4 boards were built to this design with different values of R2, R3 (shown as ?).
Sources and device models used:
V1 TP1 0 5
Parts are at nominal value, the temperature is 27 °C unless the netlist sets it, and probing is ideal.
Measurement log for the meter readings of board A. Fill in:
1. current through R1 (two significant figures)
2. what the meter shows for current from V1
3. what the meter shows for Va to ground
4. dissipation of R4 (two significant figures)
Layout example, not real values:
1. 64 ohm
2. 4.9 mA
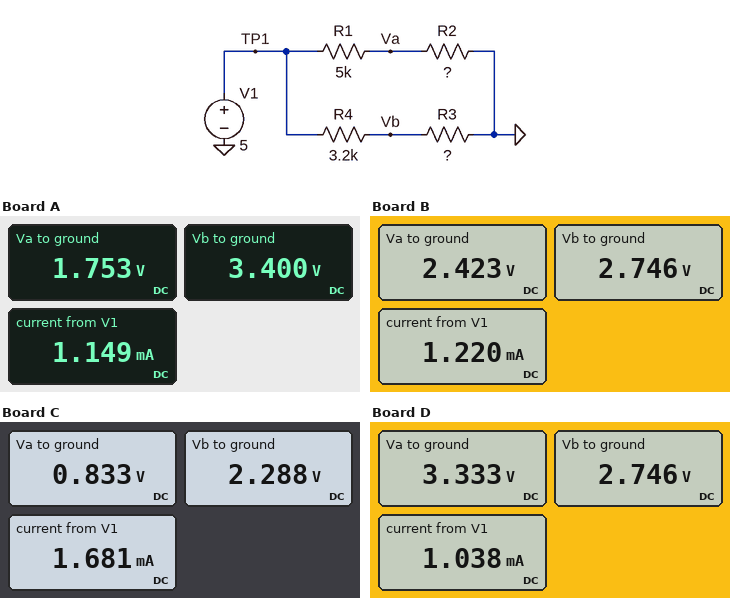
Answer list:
1. 650 µA
2. 1.149 mA
3. 1.753 V
4. 800 µW
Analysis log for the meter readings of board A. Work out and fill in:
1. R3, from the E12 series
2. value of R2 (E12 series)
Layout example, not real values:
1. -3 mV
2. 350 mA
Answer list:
1. 6.8 kΩ
2. 2.7 kΩ
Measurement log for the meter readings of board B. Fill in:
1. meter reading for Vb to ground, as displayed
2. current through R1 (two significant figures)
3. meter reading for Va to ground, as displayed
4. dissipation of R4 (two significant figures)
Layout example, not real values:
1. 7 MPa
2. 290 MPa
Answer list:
1. 2.746 V
2. 520 µA
3. 2.423 V
4. 1.6 mW
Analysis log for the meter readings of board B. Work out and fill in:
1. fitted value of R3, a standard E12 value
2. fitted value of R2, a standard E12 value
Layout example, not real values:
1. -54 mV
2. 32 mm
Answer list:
1. 3.9 kΩ
2. 4.7 kΩ
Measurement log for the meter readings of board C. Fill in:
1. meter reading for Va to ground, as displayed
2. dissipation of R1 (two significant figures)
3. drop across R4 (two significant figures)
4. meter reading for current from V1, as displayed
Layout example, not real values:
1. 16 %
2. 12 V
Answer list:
1. 0.833 V
2. 3.5 mW
3. 2.7 V
4. 1.681 mA
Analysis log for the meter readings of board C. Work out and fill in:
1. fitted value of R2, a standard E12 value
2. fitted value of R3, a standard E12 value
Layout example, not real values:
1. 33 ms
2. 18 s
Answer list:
1. 1 kΩ
2. 2.7 kΩ
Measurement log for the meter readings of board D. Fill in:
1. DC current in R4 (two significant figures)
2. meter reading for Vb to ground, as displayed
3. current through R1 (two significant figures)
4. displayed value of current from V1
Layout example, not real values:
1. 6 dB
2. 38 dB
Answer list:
1. 700 µA
2. 2.746 V
3. 330 µA
4. 1.038 mA
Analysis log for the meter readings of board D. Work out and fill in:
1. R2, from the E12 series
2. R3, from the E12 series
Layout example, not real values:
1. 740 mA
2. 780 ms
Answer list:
1. 10 kΩ
2. 3.9 kΩ
